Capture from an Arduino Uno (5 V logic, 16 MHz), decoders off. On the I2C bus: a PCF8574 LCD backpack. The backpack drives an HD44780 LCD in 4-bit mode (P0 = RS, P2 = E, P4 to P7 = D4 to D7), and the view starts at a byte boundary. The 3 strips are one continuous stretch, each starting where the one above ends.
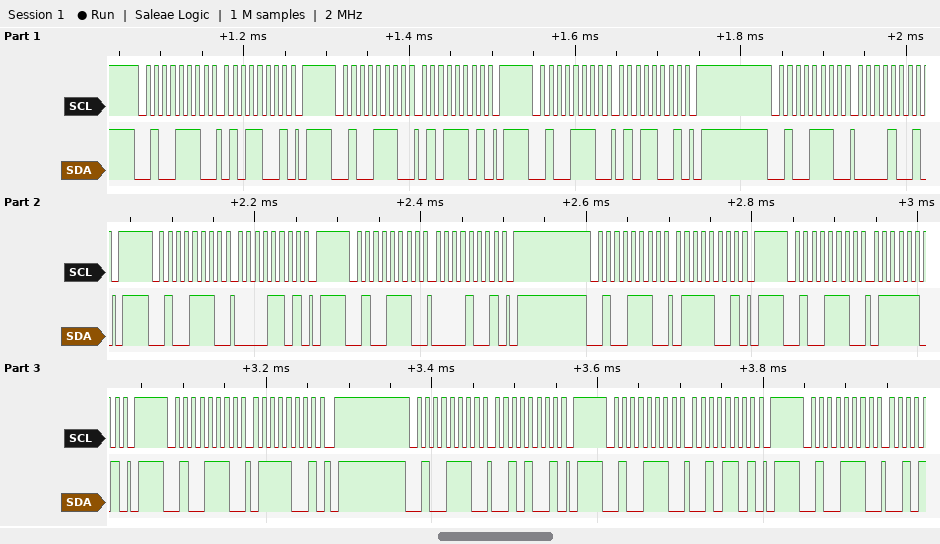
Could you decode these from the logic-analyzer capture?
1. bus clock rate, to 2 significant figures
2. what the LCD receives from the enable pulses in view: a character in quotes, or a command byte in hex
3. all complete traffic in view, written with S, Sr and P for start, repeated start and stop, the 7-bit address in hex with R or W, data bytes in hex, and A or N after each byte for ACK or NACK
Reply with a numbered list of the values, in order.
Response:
1. 100 kHz
2. 'P'
3. S 27W A 59 A P S 27W A 5D A P S 27W A 59 A P S 27W A 09 A P S 27W A 0D A P S 27W A 09 A P S 27W A 79 A P S 27W A 7D A P S 27W A 79 A P S 27W A 29 A P S 27W A 2D A P S 27W A
